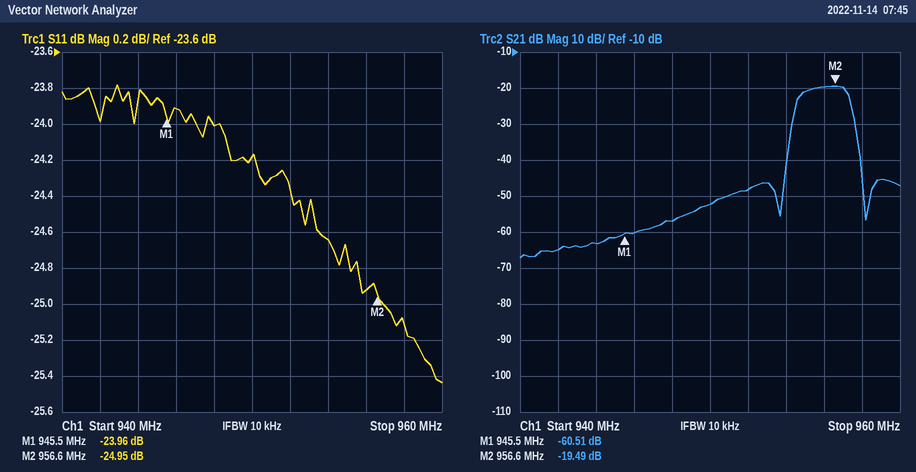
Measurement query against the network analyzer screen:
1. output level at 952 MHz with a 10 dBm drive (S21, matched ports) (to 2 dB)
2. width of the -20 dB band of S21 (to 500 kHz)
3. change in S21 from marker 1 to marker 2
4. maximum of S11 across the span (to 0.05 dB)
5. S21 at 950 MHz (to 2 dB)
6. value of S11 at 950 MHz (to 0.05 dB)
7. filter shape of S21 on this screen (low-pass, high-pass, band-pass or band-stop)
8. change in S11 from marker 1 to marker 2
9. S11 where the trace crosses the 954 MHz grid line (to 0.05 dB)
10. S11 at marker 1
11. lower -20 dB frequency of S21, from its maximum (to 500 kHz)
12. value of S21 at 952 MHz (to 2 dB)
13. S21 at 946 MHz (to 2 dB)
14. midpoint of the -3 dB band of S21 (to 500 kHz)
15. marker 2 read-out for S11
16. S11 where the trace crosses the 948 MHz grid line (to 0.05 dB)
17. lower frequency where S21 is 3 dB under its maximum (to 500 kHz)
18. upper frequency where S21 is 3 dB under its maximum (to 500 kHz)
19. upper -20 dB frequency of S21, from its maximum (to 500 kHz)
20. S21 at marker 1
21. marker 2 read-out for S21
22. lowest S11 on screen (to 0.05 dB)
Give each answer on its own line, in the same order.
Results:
-38 dBm
4.0 MHz
41.02 dB
-23.80 dB
-52 dB
-24.20 dB
band-pass
-0.99 dB
-24.65 dB
-23.96 dB
954.0 MHz
-48 dB
-60 dB
956.0 MHz
-24.95 dB
-24.00 dB
954.5 MHz
957.5 MHz
958.0 MHz
-60.51 dB
-19.49 dB
-25.45 dB
